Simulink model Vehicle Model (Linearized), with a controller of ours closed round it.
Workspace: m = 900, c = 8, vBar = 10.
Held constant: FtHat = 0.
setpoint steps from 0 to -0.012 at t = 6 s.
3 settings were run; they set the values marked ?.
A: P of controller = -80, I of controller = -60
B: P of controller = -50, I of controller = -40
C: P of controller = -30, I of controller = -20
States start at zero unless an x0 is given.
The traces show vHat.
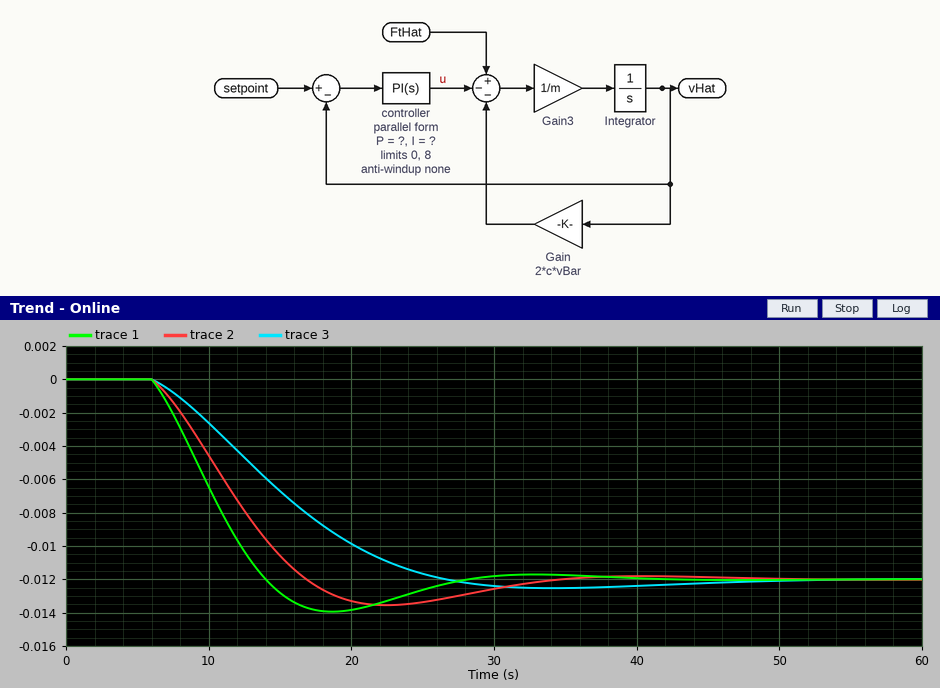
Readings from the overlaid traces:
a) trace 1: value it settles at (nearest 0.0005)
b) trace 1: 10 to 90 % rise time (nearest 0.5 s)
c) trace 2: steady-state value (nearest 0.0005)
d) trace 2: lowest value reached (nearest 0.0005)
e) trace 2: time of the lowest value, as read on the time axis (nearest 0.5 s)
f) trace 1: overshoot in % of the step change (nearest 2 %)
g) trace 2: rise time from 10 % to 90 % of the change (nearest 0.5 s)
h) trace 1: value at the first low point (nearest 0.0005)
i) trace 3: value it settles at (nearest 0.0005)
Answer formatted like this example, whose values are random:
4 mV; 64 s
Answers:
-0.0120; 6.0 s; -0.0120; -0.0135; 22.5 s; 16 %; 8.0 s; -0.0140; -0.0120
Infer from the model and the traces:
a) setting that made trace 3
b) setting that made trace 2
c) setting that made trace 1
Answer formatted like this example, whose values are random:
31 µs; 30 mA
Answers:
C; B; A
